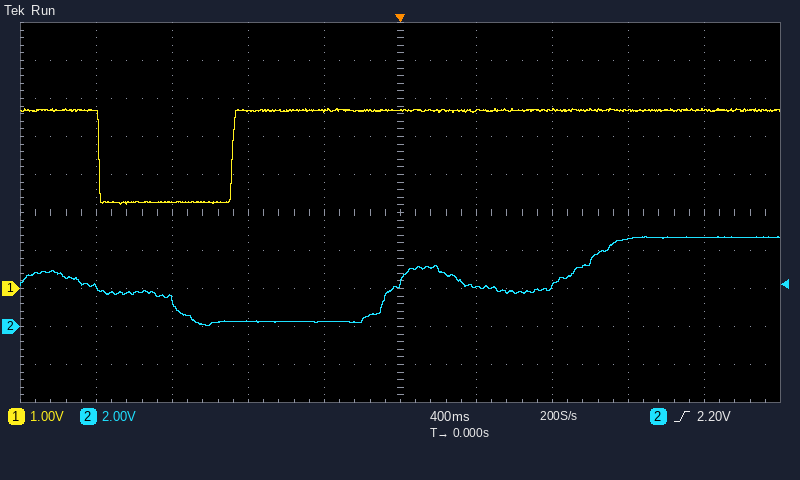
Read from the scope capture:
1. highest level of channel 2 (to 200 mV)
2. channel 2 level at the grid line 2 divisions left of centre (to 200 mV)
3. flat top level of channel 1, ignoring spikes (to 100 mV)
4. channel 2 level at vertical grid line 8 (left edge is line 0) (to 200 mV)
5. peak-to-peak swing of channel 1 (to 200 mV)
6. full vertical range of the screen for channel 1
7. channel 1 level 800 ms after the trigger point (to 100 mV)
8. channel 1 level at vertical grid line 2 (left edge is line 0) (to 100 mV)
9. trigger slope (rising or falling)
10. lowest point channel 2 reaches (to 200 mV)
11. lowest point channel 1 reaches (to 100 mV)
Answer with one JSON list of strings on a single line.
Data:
["4.8 V", "200 mV", "4.7 V", "4.6 V", "2.6 V", "10 V", "4.7 V", "2.3 V", "rising", "0.0 V", "2.2 V"]
